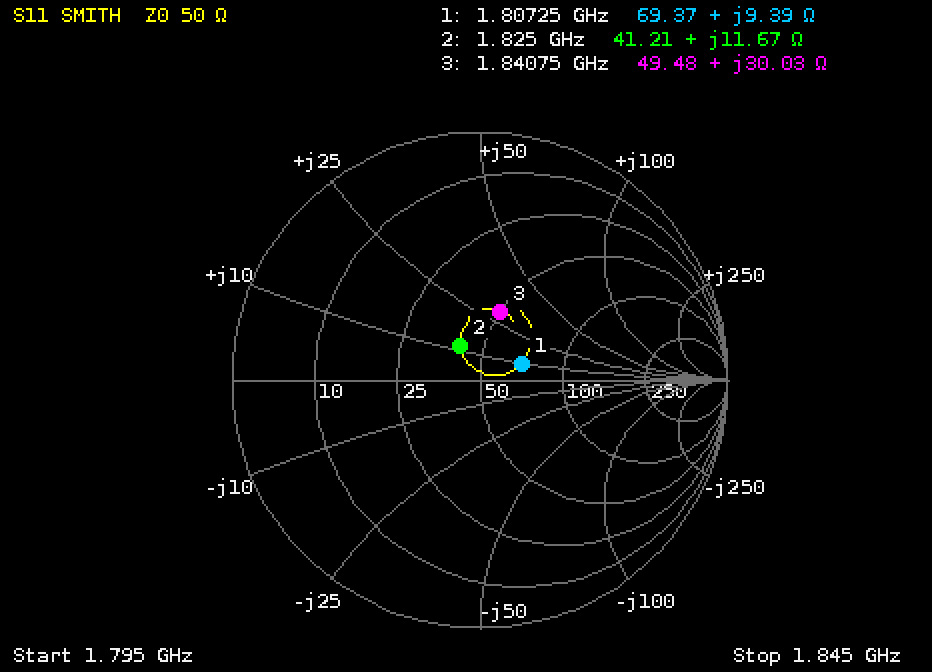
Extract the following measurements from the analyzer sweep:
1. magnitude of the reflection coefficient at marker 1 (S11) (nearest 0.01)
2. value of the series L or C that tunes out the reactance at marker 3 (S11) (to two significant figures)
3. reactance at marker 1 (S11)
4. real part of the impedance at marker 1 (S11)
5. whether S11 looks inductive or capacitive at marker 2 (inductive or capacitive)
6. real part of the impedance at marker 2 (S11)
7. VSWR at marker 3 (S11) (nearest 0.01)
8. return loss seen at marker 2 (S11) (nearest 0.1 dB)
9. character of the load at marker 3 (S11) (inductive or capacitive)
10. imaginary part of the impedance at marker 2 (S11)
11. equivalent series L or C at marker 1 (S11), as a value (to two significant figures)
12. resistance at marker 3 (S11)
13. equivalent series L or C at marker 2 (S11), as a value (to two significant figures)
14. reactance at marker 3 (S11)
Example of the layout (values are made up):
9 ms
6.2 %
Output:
0.18
2.9 pF
+9.39 Ω
69.37 Ω
inductive
41.21 Ω
1.81
16.0 dB
inductive
+11.67 Ω
830 pH
49.48 Ω
1.0 nH
+30.03 Ω
